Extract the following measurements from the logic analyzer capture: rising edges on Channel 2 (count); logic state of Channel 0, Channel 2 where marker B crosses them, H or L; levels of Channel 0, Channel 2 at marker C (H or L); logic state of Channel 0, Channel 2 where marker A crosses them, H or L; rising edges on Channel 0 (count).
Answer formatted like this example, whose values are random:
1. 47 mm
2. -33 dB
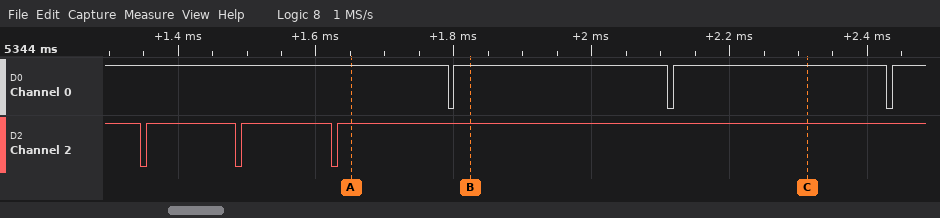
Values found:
1. 3
2. Channel 0=H, Channel 2=H
3. Channel 0=H, Channel 2=H
4. Channel 0=H, Channel 2=H
5. 3
